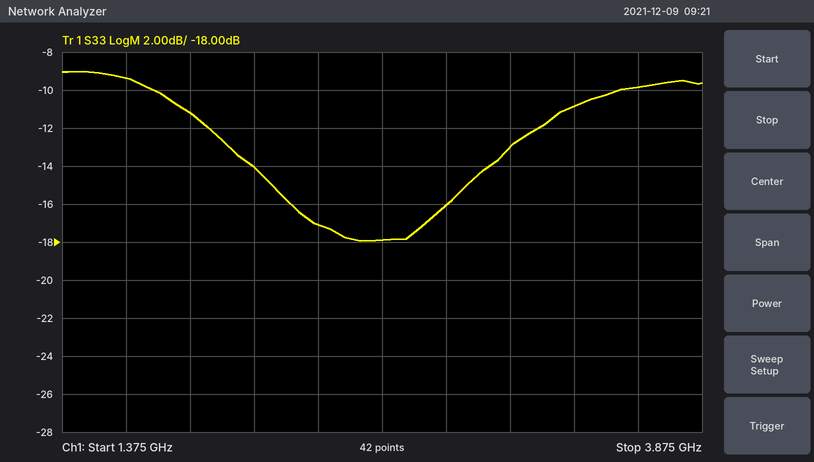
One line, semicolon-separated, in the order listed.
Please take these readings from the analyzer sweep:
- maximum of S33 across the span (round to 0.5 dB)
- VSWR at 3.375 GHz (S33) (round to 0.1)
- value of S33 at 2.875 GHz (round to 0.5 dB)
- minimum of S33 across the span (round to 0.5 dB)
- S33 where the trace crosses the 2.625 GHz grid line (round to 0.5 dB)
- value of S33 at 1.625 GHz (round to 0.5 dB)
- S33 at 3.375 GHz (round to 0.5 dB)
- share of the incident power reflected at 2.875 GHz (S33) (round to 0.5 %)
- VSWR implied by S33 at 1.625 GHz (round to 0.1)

-9.0 dB; 1.8; -16.0 dB; -18.0 dB; -18.0 dB; -9.5 dB; -11.0 dB; 2.5 %; 2.0
